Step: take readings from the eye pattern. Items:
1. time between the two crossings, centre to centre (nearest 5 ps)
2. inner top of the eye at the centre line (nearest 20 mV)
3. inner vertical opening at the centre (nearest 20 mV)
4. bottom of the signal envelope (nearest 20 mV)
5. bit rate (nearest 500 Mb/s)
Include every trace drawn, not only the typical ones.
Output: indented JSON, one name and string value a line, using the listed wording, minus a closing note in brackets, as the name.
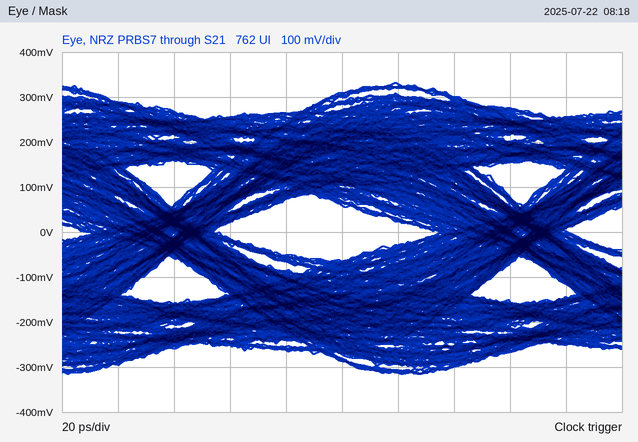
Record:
{
  "time between the two crossings, centre to centre": "125 ps",
  "inner top of the eye at the centre line": "60 mV",
  "inner vertical opening at the centre": "120 mV",
  "bottom of the signal envelope": "-320 mV",
  "bit rate": "8.0 Gb/s"
}
